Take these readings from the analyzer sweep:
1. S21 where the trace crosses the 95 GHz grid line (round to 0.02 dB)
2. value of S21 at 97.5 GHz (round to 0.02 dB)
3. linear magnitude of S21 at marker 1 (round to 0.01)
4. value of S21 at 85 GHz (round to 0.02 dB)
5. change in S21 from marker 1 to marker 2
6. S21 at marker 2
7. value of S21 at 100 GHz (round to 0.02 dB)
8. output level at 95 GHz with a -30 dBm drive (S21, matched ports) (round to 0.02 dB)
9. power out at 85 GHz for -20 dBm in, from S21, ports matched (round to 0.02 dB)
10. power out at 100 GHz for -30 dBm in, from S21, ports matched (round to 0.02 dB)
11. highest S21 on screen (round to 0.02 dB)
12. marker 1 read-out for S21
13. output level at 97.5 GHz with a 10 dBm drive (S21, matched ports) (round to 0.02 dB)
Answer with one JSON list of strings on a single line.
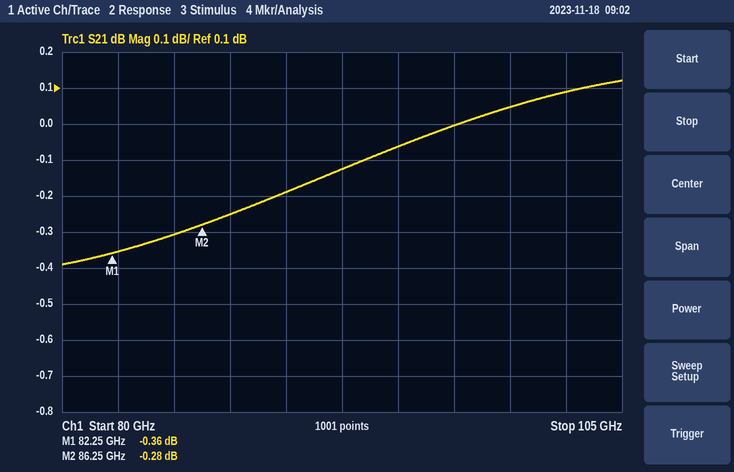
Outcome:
["-0.06 dB", "0.00 dB", "0.96", "-0.30 dB", "0.08 dB", "-0.28 dB", "0.04 dB", "-30.06 dBm", "-20.30 dBm", "-29.96 dBm", "0.12 dB", "-0.36 dB", "10.00 dBm"]
